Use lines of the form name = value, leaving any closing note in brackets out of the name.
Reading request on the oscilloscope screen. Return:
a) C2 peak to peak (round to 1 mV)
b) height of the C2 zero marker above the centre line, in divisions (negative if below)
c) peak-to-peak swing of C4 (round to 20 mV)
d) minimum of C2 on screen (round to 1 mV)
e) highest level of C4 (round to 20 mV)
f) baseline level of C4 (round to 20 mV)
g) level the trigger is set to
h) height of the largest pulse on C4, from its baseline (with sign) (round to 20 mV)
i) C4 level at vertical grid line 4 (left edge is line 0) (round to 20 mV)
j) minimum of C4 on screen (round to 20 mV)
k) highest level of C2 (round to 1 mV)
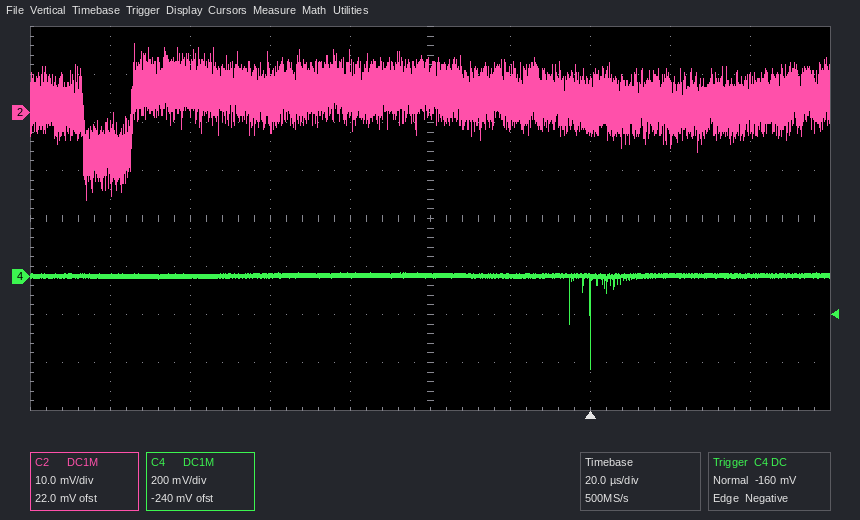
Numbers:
C2 peak to peak = 32 mV
height of the C2 zero marker above the centre line, in divisions = +2.2 div
peak-to-peak swing of C4 = 400 mV
minimum of C2 on screen = -18 mV
highest level of C4 = 20 mV
baseline level of C4 = 0 mV
level the trigger is set to = -160 mV
height of the largest pulse on C4, from its baseline (with sign) = -380 mV
C4 level at vertical grid line 4 (left edge is line 0) = 0 mV
minimum of C4 on screen = -380 mV
highest level of C2 = 14 mV
